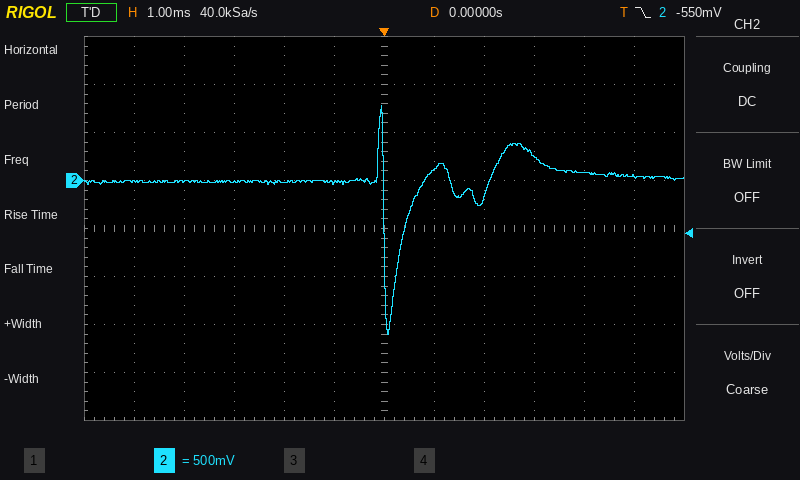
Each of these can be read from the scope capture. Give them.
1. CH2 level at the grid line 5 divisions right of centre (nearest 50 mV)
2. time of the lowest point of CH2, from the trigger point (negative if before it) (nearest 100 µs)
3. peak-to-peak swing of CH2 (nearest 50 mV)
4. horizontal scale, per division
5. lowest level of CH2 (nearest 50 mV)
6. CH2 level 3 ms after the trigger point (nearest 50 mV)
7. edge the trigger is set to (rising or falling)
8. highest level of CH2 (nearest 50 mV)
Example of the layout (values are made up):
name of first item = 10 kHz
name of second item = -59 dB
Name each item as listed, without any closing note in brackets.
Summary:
CH2 level at the grid line 5 divisions right of centre = 50 mV
time of the lowest point of CH2, from the trigger point (negative if before it) = +100 µs
peak-to-peak swing of CH2 = 2.40 V
horizontal scale, per division = 1 ms
lowest level of CH2 = -1.60 V
CH2 level 3 ms after the trigger point = 250 mV
edge the trigger is set to = falling
highest level of CH2 = 800 mV
